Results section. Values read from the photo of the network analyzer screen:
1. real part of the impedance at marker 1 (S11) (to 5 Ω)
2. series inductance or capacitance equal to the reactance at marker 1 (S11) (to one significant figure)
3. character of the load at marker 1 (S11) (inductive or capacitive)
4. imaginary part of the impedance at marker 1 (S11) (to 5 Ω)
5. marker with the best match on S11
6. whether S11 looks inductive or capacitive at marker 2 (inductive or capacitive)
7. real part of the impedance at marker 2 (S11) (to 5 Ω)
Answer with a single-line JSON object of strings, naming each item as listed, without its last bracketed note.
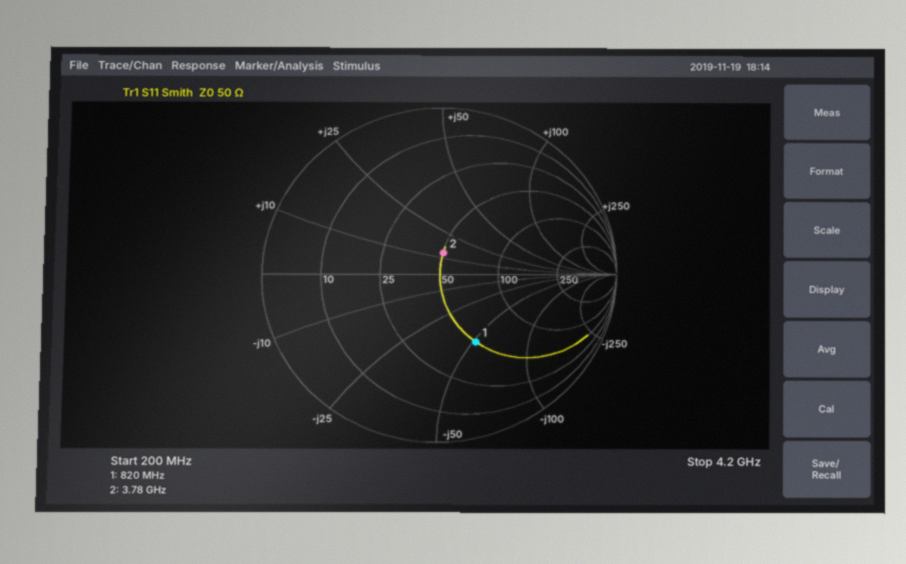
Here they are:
{"real part of the impedance at marker 1 (S11)": "50 Ω", "series inductance or capacitance equal to the reactance at marker 1 (S11)": "4 pF", "character of the load at marker 1 (S11)": "capacitive", "imaginary part of the impedance at marker 1 (S11)": "-50 Ω", "marker with the best match on S11": "marker 2", "whether S11 looks inductive or capacitive at marker 2": "inductive", "real part of the impedance at marker 2 (S11)": "50 Ω"}
